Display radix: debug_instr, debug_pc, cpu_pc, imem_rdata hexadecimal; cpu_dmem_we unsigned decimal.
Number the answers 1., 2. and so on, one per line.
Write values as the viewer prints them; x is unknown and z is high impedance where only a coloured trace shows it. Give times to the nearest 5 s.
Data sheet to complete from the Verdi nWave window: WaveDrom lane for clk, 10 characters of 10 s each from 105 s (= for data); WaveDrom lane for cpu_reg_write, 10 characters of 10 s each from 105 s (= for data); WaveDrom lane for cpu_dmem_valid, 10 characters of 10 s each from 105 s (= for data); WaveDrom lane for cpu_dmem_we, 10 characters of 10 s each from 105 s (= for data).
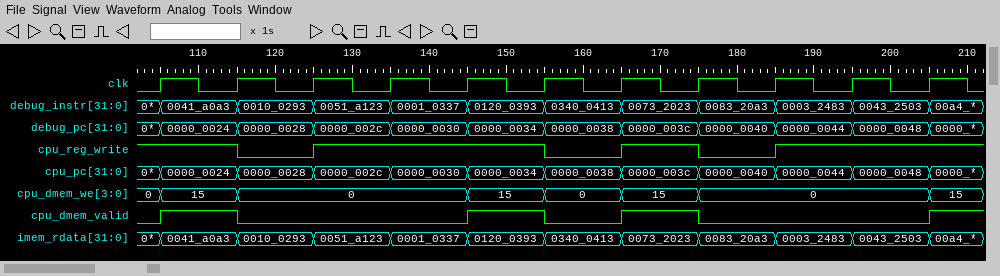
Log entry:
1. {name: 'clk', wave: 'p.........'}
2. {name: 'cpu_reg_write', wave: '101..0101.'}
3. {name: 'cpu_dmem_valid', wave: '10..1010..'}
4. {name: 'cpu_dmem_we', wave: '==..====..', data: '15 0 15 0 15 0'}
